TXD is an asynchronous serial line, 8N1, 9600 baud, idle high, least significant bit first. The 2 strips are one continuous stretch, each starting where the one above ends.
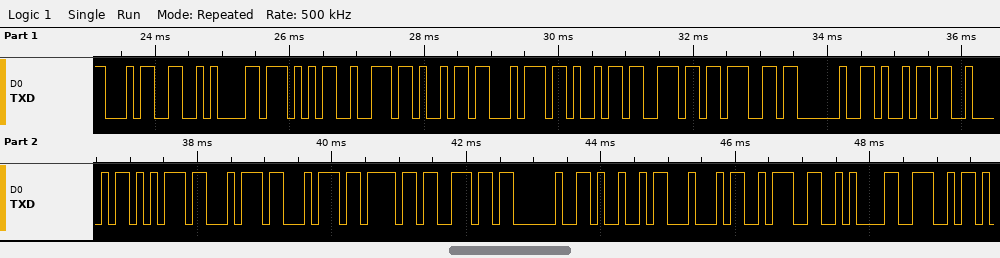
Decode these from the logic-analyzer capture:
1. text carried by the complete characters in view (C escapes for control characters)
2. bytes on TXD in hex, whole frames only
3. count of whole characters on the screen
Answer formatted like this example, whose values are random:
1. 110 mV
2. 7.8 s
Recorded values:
1. "4\nWriting iButton ID:\nN"
2. 34 0A 57 72 69 74 69 6E 67 20 69 42 75 74 74 6F 6E 20 49 44 3A 0A 4E
3. 23
